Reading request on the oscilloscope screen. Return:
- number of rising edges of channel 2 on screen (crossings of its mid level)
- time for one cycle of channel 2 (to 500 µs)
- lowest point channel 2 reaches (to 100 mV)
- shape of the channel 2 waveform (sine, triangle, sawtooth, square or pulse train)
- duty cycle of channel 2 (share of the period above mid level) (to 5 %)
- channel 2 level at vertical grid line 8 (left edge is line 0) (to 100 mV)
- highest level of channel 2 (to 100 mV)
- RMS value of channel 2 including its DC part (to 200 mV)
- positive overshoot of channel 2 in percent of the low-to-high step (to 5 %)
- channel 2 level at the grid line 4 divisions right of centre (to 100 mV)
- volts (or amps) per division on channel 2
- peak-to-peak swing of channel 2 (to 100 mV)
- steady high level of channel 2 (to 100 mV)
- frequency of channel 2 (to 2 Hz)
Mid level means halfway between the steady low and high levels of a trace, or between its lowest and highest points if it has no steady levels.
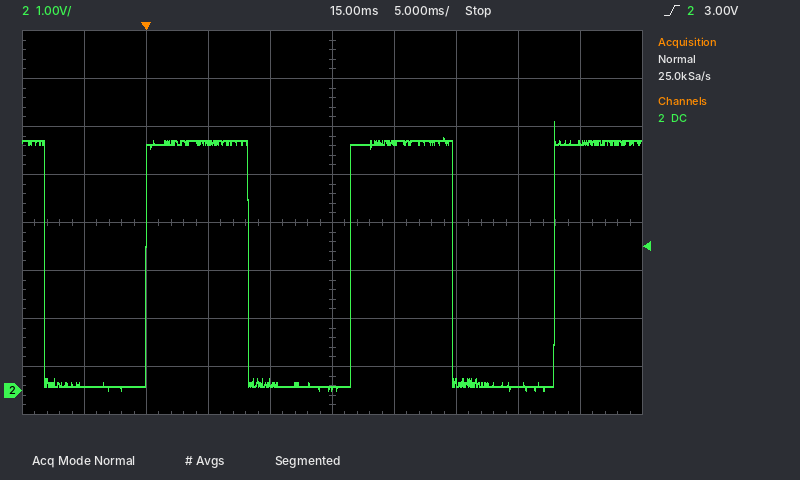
3
16.5 ms
0.0 V
square
50 %
100 mV
5.6 V
3.6 V
10 %
5.2 V
1 V
5.6 V
5.2 V
60 Hz
